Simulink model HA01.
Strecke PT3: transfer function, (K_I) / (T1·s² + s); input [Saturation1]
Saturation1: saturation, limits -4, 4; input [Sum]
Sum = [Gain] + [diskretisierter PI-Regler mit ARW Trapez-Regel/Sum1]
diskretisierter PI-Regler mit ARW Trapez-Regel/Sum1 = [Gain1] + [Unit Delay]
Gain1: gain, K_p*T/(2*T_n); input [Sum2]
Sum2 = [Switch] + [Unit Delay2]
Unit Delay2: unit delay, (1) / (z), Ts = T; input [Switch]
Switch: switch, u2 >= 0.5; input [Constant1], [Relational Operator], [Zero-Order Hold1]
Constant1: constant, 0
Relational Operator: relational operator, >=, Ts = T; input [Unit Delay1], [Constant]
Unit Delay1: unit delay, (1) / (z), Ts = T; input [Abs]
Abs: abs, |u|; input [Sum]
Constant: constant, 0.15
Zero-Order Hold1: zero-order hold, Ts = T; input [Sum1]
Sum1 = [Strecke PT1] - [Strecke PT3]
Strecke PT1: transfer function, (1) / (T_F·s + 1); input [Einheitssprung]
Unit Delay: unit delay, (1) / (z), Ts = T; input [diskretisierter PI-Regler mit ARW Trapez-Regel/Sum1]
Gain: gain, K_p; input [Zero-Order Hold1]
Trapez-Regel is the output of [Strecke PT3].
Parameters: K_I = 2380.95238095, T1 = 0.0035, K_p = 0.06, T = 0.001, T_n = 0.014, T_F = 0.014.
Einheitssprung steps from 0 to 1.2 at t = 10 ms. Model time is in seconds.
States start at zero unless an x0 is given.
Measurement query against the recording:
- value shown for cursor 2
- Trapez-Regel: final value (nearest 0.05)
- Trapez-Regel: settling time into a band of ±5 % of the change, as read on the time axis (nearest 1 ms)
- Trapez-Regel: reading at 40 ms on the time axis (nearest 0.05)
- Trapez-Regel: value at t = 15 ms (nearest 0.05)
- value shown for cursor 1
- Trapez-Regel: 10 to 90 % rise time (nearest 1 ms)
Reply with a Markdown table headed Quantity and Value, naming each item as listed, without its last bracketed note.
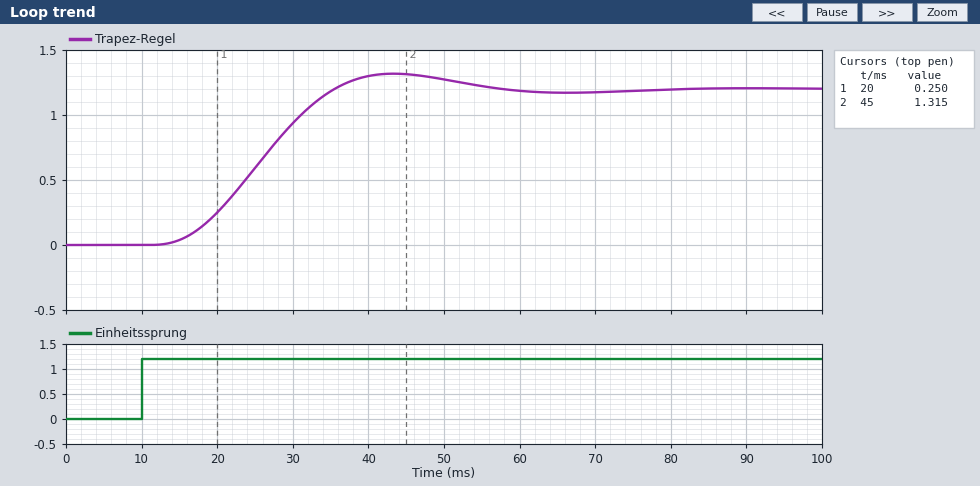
| Quantity | Value |
|---|---|
| value shown for cursor 2 | 1.315 |
| Trapez-Regel: final value | 1.20 |
| Trapez-Regel: settling time into a band of ±5 % of the change, as read on the time axis | 51 ms |
| Trapez-Regel: reading at 40 ms on the time axis | 1.30 |
| Trapez-Regel: value at t = 15 ms | 0.05 |
| value shown for cursor 1 | 0.250 |
| Trapez-Regel: 10 to 90 % rise time | 15 ms |
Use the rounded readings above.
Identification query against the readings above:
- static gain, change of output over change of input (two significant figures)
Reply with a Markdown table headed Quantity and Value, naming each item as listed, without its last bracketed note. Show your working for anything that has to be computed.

| Quantity | Value |
|---|---|
| static gain, change of output over change of input | (1.2 - 0) / (1.2 - 0) = 1.0 |
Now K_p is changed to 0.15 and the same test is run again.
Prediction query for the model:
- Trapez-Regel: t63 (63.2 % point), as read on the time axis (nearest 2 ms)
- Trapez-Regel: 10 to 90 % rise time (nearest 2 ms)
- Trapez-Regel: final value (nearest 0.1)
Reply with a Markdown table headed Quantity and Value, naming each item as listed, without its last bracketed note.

| Quantity | Value |
|---|---|
| Trapez-Regel: t63 (63.2 % point), as read on the time axis | 22 ms |
| Trapez-Regel: 10 to 90 % rise time | 26 ms |
| Trapez-Regel: final value | 1.2 |
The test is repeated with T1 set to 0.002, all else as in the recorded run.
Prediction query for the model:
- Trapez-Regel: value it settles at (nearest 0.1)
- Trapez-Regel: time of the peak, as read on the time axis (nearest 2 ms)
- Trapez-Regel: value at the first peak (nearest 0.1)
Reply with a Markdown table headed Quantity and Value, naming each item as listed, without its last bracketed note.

| Quantity | Value |
|---|---|
| Trapez-Regel: value it settles at | 1.2 |
| Trapez-Regel: time of the peak, as read on the time axis | 46 ms |
| Trapez-Regel: value at the first peak | 1.3 |
